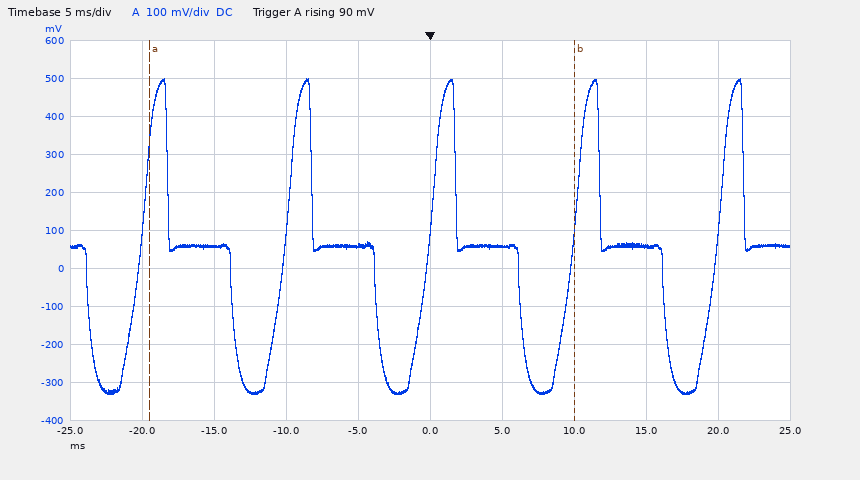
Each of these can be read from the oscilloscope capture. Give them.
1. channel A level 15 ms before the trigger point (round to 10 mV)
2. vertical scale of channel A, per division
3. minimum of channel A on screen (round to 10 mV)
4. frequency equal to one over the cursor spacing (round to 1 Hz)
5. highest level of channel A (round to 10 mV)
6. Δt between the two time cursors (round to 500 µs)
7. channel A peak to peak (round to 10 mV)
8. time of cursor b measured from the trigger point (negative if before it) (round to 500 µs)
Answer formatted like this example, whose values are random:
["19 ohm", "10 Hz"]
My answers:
["60 mV", "100 mV", "-330 mV", "34 Hz", "500 mV", "29.5 ms", "830 mV", "+10.0 ms"]
